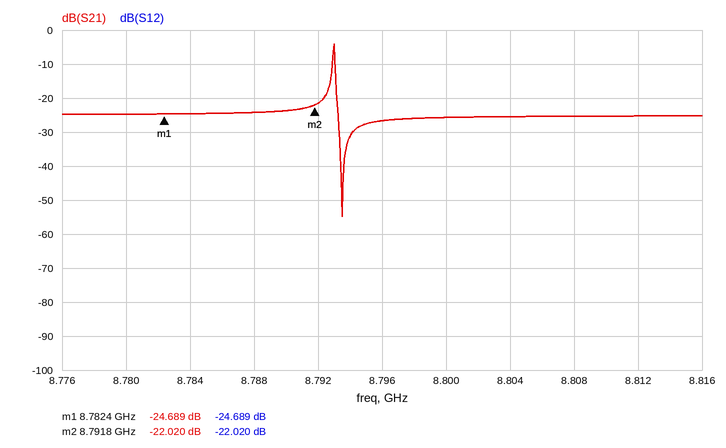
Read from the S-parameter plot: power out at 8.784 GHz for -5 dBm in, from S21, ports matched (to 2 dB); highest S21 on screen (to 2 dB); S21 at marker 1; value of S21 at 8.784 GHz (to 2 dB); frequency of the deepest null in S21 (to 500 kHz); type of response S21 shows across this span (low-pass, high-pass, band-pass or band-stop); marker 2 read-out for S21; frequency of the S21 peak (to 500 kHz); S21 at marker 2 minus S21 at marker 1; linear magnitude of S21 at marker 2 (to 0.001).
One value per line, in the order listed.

-30 dBm
-4 dB
-24.689 dB
-24 dB
8.7935 GHz
band-pass
-22.020 dB
8.7930 GHz
2.669 dB
0.079
